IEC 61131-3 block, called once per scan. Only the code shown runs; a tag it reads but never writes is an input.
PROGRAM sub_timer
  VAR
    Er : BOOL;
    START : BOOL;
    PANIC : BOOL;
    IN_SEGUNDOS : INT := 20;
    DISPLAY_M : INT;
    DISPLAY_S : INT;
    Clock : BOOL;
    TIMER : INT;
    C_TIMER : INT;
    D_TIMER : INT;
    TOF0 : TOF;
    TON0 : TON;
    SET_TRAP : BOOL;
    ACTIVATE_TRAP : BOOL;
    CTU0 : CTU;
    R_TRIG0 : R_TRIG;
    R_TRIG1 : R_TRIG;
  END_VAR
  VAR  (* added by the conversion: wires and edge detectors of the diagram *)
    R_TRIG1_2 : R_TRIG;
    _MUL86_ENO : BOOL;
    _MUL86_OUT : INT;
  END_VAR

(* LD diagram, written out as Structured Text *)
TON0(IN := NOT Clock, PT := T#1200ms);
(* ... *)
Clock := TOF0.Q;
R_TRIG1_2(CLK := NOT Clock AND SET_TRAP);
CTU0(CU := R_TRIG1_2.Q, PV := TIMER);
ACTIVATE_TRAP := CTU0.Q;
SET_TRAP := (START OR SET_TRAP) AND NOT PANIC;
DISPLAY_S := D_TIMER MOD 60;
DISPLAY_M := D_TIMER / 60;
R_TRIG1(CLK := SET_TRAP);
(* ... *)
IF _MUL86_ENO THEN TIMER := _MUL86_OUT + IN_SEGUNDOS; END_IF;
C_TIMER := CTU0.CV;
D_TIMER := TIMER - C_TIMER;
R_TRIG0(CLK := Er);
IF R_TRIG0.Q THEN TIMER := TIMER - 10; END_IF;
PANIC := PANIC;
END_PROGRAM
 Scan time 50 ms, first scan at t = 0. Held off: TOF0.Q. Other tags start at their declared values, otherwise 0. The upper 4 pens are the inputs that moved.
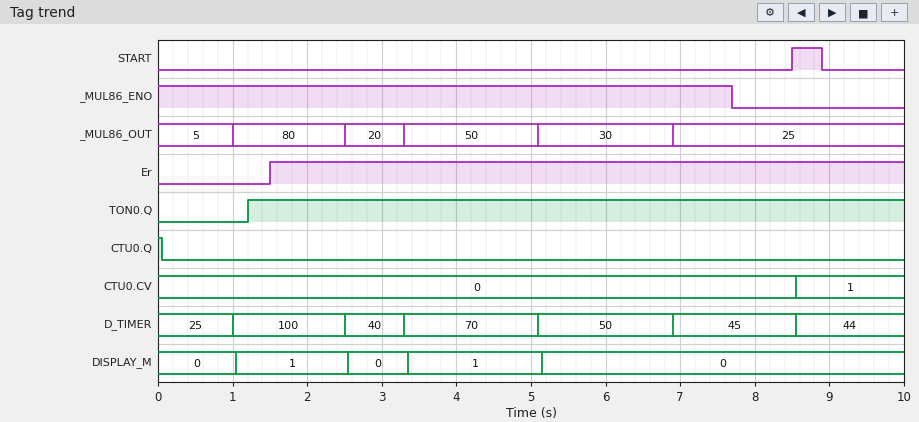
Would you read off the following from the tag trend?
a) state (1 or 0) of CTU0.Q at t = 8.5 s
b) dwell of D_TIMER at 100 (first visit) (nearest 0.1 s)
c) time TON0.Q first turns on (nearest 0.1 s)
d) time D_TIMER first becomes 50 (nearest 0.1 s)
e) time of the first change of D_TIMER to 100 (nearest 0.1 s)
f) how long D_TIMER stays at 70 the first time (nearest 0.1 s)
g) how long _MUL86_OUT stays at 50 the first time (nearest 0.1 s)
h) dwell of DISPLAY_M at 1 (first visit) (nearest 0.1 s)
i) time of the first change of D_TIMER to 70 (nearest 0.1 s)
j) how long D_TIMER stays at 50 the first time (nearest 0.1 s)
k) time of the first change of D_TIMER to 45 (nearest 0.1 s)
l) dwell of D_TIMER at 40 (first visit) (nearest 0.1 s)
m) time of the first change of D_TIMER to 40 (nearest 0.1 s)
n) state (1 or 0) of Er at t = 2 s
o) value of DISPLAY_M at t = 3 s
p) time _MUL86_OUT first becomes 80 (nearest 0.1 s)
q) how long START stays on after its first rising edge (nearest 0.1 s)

0
1.5 s
1.2 s
5.1 s
1.0 s
1.8 s
1.8 s
1.5 s
3.3 s
1.8 s
6.9 s
0.8 s
2.5 s
1
0
1.0 s
0.4 s
